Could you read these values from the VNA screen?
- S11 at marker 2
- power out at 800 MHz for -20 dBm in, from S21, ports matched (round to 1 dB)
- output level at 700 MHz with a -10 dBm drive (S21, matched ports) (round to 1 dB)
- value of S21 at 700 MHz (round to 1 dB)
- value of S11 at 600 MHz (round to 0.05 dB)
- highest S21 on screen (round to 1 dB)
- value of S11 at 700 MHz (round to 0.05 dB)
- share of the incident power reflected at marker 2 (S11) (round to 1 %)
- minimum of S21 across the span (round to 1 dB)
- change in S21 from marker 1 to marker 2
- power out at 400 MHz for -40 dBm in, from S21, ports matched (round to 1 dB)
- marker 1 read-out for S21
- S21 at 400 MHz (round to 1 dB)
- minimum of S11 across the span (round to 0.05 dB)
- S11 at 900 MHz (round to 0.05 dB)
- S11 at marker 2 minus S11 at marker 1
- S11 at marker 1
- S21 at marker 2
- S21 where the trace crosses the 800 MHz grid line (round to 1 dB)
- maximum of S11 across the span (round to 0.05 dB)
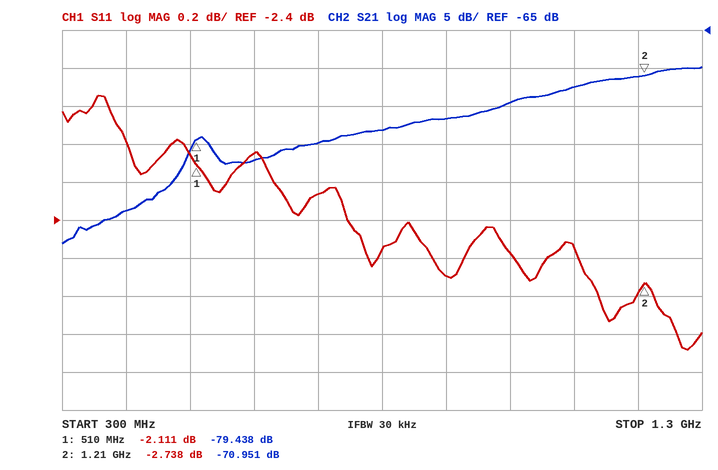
-2.738 dB
-98 dBm
-90 dBm
-80 dB
-2.05 dB
-70 dB
-2.25 dB
53 %
-93 dB
8.487 dB
-129 dBm
-79.438 dB
-89 dB
-3.10 dB
-2.70 dB
-0.627 dB
-2.111 dB
-70.951 dB
-78 dB
-1.75 dB
